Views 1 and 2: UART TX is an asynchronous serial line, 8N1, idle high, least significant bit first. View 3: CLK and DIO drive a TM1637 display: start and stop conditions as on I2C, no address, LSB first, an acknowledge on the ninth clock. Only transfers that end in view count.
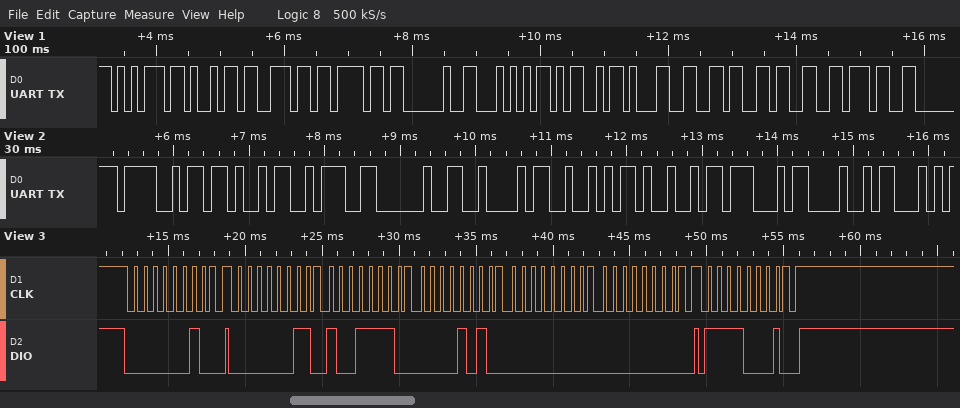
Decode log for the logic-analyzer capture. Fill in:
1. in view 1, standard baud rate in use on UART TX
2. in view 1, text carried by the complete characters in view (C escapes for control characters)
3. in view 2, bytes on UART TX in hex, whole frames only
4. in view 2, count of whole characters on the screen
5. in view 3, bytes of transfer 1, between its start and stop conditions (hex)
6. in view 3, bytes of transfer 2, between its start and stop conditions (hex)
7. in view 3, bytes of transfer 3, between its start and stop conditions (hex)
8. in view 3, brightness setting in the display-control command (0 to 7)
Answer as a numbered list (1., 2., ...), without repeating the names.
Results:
1. 9600 baud
2. "uino TM1637"
3. 4F 4B 3A 20 42 52 49 47 48
4. 9
5. 40
6. C0 79 50 00 00
7. 8F
8. 7
